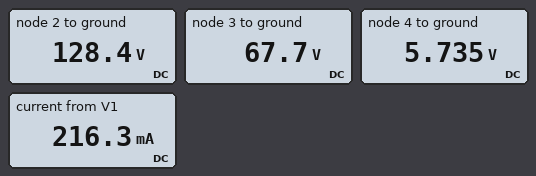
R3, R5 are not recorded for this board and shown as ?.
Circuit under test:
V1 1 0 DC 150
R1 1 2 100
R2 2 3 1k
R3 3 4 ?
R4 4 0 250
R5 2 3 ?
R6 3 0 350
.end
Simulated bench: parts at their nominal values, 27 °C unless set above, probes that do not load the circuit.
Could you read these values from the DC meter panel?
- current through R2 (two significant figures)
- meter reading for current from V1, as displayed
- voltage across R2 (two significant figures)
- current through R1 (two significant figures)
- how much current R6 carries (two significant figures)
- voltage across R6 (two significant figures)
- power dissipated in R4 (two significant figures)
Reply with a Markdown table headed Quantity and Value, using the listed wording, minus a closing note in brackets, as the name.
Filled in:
| Quantity | Value |
|---|---|
| current through R2 | 61 mA |
| meter reading for current from V1, as displayed | 216.3 mA |
| voltage across R2 | 61 V |
| current through R1 | 220 mA |
| how much current R6 carries | 190 mA |
| voltage across R6 | 68 V |
| power dissipated in R4 | 130 mW |
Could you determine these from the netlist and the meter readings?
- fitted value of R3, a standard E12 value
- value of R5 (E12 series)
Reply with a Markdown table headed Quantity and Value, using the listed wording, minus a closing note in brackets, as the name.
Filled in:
| Quantity | Value |
|---|---|
| fitted value of R3, a standard E12 value | 2.7 kΩ |
| value of R5 | 390 Ω |
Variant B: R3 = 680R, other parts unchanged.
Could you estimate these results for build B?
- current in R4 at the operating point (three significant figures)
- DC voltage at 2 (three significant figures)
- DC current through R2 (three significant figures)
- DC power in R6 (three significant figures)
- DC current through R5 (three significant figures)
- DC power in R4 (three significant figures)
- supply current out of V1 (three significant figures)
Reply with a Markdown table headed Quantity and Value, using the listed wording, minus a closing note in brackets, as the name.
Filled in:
| Quantity | Value |
|---|---|
| current in R4 at the operating point | 64.6 mA |
| DC voltage at 2 | 126 V |
| DC current through R2 | 66.3 mA |
| DC power in R6 | 10.3 W |
| DC current through R5 | 170 mA |
| DC power in R4 | 1.04 W |
| supply current out of V1 | 236 mA |
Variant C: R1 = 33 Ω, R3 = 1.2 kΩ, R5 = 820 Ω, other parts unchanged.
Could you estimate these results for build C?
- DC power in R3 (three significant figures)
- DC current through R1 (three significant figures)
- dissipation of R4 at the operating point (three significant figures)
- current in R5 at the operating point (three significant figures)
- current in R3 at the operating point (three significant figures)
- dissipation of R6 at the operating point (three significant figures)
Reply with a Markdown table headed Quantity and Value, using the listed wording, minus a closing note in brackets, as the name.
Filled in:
| Quantity | Value |
|---|---|
| DC power in R3 | 1.74 W |
| DC current through R1 | 196 mA |
| dissipation of R4 at the operating point | 363 mW |
| current in R5 at the operating point | 108 mA |
| current in R3 at the operating point | 38.1 mA |
| dissipation of R6 at the operating point | 8.72 W |
